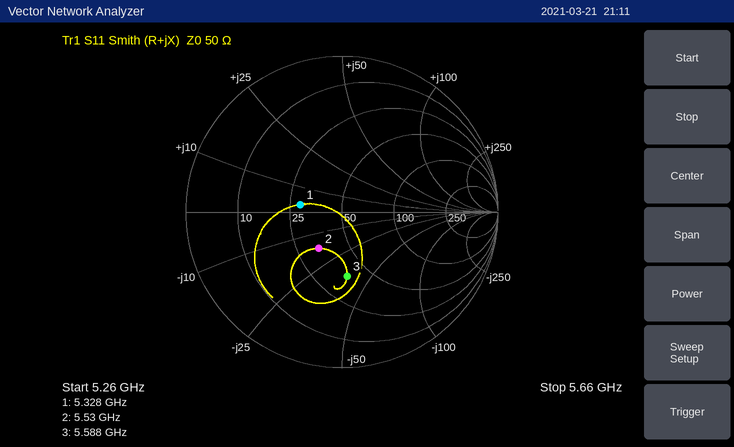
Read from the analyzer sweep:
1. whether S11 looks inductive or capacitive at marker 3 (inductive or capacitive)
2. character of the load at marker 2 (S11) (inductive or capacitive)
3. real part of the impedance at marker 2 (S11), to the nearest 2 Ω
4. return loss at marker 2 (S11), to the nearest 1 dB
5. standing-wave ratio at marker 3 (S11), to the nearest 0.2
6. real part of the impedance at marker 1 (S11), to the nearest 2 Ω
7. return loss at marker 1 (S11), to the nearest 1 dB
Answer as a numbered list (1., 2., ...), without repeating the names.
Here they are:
1. capacitive
2. capacitive
3. 34 Ω
4. 11 dB
5. 2.4
6. 28 Ω
7. 11 dB
